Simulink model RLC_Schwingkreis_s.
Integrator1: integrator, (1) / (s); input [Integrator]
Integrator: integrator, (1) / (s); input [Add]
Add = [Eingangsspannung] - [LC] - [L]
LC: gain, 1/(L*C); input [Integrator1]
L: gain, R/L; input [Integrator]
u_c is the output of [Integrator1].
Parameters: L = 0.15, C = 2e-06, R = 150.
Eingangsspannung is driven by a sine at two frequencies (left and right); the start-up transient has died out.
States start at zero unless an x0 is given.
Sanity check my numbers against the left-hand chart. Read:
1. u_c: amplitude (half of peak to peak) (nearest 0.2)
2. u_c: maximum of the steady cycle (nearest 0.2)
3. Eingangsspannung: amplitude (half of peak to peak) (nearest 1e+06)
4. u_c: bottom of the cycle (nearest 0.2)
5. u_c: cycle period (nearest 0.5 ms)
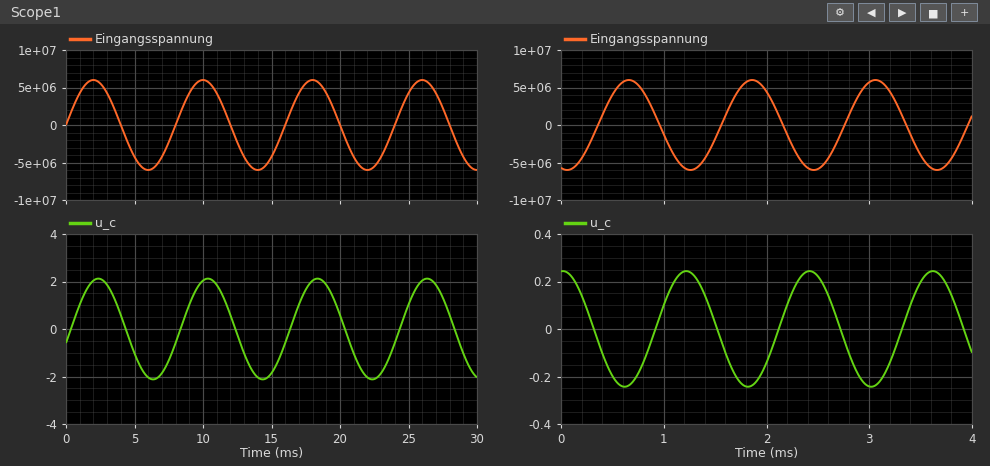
2.2
2.2
6000000
-2.2
8.0 ms
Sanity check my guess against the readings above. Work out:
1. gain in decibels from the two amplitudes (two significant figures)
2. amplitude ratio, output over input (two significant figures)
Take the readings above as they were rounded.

-130 dB
0.00000037
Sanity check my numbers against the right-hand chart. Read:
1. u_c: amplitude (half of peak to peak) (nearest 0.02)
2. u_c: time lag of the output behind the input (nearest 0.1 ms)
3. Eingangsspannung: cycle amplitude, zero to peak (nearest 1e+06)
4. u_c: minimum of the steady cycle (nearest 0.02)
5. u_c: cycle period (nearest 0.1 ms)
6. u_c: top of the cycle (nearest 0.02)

0.24
0.6 ms
6000000
-0.24
1.2 ms
0.24
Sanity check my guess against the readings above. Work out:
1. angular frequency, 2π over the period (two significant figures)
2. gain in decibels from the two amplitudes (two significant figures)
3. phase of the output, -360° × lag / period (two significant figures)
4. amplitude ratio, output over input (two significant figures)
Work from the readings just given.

5.2 rad/ms
-150 dB
-180°
0.000000040
